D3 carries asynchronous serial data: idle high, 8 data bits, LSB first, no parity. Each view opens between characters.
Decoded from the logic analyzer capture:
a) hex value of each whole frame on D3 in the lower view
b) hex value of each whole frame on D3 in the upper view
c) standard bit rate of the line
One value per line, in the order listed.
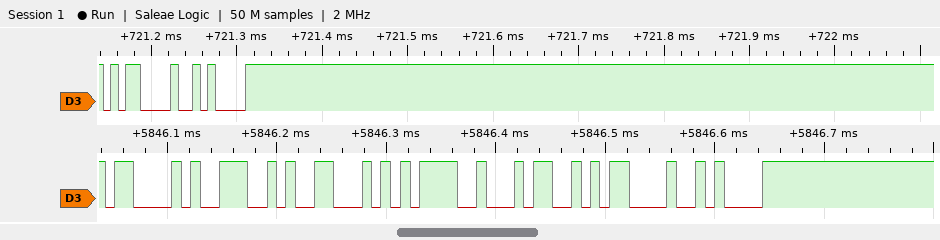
43, 4E, 46, 3D, 34, 0D, 0A
0D, 0A
115200 baud
